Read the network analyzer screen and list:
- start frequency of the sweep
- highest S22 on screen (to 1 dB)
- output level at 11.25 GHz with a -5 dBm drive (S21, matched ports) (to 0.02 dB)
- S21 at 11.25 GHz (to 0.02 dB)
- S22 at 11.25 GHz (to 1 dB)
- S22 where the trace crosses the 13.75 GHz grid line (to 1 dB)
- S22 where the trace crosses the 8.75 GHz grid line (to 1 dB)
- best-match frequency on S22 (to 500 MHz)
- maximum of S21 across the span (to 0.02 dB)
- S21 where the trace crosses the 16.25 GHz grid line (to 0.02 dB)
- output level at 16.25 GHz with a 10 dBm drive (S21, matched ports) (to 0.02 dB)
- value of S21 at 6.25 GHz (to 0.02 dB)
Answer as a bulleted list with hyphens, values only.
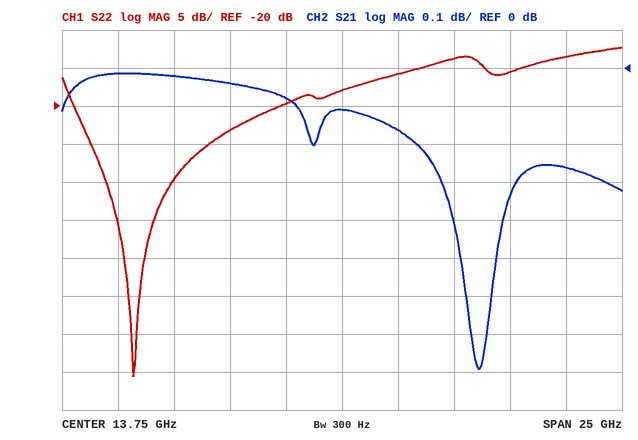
- 1.25 GHz
- -12 dB
- -5.08 dBm
- -0.08 dB
- -20 dB
- -18 dB
- -23 dB
- 4.5 GHz
- -0.02 dB
- -0.16 dB
- 9.84 dBm
- -0.02 dB
